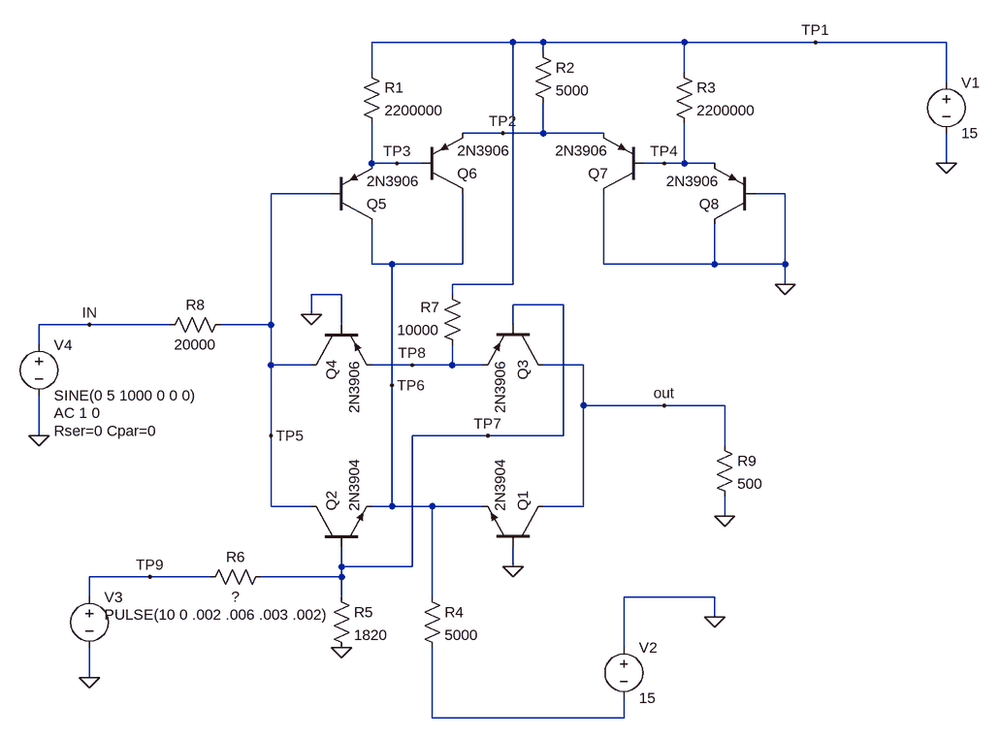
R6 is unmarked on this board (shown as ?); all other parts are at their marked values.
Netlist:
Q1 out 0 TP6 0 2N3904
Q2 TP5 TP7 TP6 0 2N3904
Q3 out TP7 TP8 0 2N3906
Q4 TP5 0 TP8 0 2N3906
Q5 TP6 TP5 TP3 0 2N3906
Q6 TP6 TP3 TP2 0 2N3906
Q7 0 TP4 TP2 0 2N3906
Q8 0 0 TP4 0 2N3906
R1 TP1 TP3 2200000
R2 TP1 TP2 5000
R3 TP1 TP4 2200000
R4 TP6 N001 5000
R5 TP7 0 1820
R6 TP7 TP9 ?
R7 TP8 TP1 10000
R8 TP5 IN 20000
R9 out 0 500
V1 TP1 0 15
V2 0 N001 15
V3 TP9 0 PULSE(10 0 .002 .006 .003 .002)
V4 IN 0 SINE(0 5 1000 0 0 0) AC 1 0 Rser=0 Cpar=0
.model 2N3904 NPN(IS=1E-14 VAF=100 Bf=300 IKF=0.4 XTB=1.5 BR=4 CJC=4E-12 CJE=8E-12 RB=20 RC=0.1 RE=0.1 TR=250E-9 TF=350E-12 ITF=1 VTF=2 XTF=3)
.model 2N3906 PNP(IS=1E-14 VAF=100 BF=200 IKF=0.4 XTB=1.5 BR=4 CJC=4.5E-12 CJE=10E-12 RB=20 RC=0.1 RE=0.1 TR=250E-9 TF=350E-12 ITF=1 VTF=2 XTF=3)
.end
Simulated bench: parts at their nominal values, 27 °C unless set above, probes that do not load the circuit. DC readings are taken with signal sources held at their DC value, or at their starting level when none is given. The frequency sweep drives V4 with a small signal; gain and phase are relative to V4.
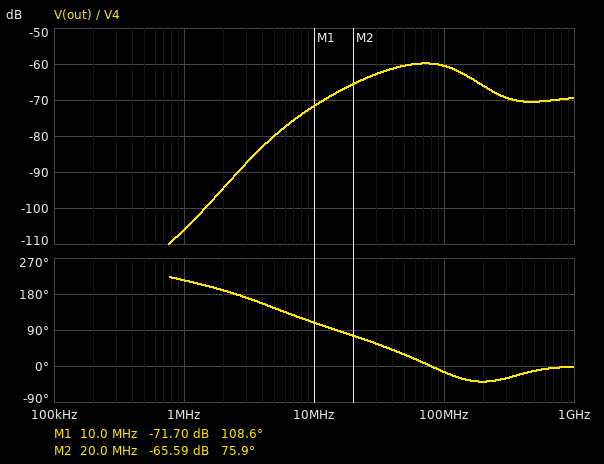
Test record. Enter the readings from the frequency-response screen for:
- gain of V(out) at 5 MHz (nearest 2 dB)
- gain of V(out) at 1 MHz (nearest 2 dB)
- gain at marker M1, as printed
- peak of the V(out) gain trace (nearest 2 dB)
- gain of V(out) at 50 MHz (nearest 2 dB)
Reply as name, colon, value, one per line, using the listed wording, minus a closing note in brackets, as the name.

gain of V(out) at 5 MHz: -80 dB
gain of V(out) at 1 MHz: -106 dB
gain at marker M1, as printed: -71.70 dB
peak of the V(out) gain trace: -60 dB
gain of V(out) at 50 MHz: -60 dB
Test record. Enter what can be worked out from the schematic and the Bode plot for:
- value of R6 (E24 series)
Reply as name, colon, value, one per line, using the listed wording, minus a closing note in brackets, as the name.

value of R6: 36 kΩ
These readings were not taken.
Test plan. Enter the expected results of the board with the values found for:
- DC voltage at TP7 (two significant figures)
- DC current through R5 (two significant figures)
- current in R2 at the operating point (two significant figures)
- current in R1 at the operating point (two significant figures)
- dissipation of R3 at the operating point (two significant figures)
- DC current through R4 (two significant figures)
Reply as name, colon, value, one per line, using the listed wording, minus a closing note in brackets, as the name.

DC voltage at TP7: 470 mV
DC current through R5: 260 µA
current in R2 at the operating point: 2.8 mA
current in R1 at the operating point: 6.6 µA
dissipation of R3 at the operating point: 95 µW
DC current through R4: 3.0 mA
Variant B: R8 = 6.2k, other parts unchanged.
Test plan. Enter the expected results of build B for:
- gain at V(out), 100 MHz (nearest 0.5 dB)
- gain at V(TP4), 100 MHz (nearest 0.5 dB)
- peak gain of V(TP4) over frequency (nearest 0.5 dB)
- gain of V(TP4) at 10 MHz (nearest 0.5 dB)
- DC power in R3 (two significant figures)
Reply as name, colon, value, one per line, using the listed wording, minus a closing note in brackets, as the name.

gain at V(out), 100 MHz: -50.5 dB
gain at V(TP4), 100 MHz: -47.5 dB
peak gain of V(TP4) over frequency: -45.0 dB
gain of V(TP4) at 10 MHz: -45.5 dB
DC power in R3: 95 µW
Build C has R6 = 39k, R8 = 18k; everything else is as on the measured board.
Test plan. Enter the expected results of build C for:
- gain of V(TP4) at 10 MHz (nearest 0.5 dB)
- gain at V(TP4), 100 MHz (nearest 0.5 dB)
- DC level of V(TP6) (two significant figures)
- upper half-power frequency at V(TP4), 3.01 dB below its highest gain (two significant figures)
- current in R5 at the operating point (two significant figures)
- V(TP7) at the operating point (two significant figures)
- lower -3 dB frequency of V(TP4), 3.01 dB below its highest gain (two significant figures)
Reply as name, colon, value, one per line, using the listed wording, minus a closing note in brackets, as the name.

gain of V(TP4) at 10 MHz: -54.5 dB
gain at V(TP4), 100 MHz: -55.5 dB
DC level of V(TP6): -230 mV
upper half-power frequency at V(TP4), 3.01 dB below its highest gain: 120 MHz
current in R5 at the operating point: 240 µA
V(TP7) at the operating point: 440 mV
lower -3 dB frequency of V(TP4), 3.01 dB below its highest gain: 3.9 MHz
